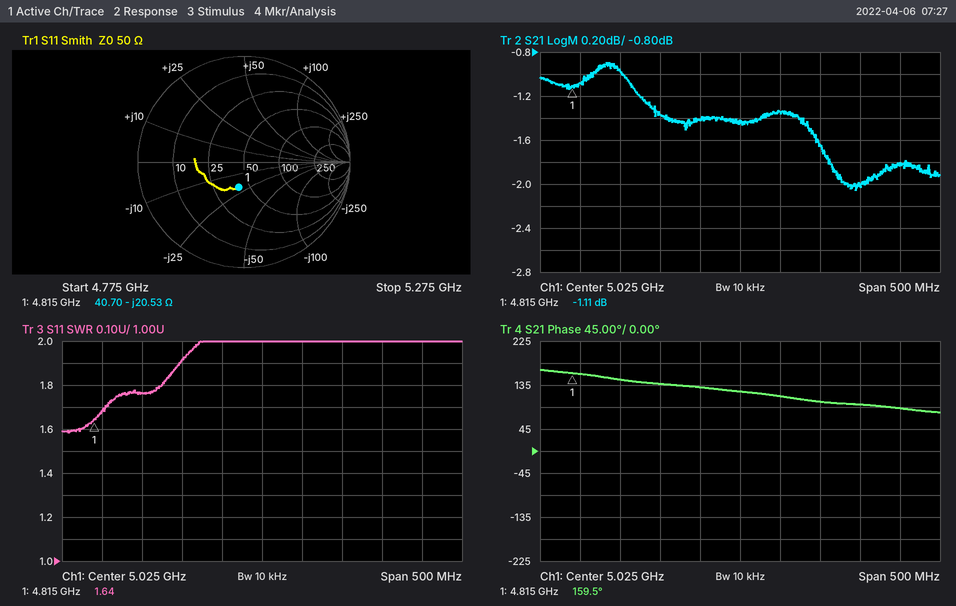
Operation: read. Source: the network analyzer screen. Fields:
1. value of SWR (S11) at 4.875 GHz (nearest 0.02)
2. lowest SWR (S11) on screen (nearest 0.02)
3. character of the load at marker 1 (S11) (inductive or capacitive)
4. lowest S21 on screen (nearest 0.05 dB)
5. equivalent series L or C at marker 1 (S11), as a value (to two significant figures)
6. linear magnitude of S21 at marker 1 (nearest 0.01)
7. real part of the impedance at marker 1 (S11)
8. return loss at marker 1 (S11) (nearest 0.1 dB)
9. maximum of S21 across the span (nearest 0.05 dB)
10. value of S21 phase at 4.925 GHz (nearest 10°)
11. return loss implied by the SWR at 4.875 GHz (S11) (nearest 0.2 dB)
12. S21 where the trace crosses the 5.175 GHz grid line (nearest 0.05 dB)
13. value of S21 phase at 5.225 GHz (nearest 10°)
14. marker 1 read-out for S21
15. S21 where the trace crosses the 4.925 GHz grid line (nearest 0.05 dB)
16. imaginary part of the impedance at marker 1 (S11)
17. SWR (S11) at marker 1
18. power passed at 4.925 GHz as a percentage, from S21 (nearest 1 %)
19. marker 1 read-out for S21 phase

1.76
1.58
capacitive
-2.05 dB
1.6 pF
0.88
40.70 Ω
12.3 dB
-0.90 dB
140°
11.2 dB
-2.00 dB
90°
-1.11 dB
-1.35 dB
-20.53 Ω
1.64
73 %
159.5°
